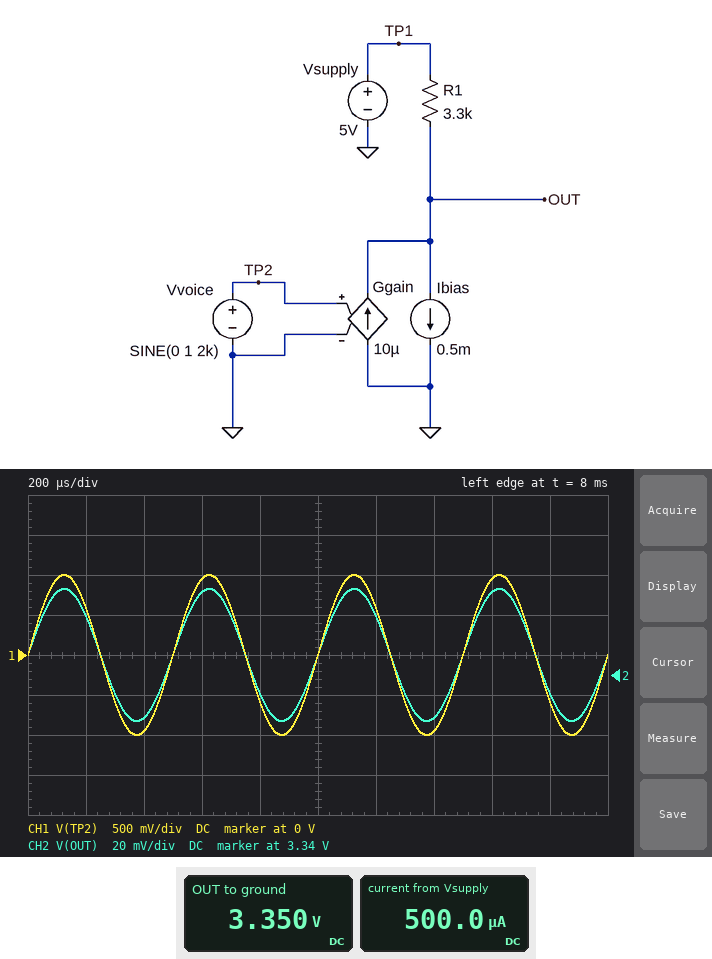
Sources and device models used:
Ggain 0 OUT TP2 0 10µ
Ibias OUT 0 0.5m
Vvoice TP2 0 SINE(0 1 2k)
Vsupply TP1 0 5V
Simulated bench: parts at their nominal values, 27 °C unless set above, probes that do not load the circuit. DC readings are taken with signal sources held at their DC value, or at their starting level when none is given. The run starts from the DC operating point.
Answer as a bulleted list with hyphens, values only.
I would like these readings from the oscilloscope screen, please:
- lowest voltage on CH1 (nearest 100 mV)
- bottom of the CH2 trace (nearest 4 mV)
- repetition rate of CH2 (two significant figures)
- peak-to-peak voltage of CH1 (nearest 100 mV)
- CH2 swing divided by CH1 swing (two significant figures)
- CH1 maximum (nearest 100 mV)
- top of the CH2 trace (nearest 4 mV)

- -1.0 V
- 3.316 V
- 2.0 kHz
- 2.0 V
- 0.033
- 1.0 V
- 3.384 V
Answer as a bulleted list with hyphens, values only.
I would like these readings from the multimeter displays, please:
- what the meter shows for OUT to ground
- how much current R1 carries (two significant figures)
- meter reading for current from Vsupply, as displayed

- 3.350 V
- 500 µA
- 500.0 µA
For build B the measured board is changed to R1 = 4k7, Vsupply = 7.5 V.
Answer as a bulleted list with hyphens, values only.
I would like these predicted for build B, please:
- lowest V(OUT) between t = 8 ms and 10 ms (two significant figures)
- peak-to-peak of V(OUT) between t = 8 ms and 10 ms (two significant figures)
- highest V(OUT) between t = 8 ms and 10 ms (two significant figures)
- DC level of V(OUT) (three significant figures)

- 5.1 V
- 94 mV
- 5.2 V
- 5.15 V
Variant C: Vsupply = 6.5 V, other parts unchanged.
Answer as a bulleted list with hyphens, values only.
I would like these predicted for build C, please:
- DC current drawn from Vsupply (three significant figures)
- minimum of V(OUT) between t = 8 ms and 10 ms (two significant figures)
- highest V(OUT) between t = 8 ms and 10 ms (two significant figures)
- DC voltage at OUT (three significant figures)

- 500 µA
- 4.8 V
- 4.9 V
- 4.85 V
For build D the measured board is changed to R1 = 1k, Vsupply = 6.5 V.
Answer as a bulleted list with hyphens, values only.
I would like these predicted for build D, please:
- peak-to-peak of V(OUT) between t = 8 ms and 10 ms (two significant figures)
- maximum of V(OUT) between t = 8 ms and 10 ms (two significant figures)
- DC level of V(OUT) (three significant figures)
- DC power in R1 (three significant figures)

- 20 mV
- 6.0 V
- 6.00 V
- 250 µW
